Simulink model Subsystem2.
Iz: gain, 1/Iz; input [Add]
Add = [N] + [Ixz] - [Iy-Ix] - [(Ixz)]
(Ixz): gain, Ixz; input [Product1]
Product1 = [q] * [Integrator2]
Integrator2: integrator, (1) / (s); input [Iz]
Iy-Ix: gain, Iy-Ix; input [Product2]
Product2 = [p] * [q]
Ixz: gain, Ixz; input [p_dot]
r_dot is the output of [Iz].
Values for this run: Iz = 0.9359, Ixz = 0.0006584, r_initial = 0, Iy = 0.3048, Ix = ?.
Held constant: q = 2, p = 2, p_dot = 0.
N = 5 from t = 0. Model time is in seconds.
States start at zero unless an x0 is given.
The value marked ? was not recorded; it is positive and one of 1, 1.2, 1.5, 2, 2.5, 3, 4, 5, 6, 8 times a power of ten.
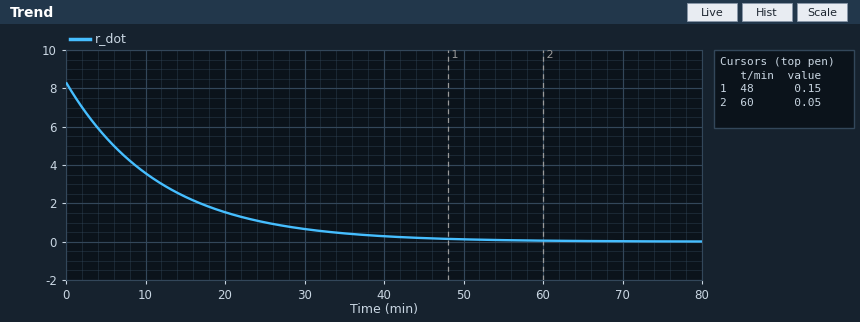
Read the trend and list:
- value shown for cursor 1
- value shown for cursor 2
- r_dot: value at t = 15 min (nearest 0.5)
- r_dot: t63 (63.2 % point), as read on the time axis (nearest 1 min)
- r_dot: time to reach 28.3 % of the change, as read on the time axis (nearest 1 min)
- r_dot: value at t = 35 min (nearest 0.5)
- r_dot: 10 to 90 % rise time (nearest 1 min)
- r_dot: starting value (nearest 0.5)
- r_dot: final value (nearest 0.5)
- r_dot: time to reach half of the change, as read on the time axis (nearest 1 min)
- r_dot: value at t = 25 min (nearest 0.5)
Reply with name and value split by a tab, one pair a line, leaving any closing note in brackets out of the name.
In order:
value shown for cursor 1	0.15
value shown for cursor 2	0.05
r_dot: value at t = 15 min	2.5
r_dot: t63 (63.2 % point), as read on the time axis	12 min
r_dot: time to reach 28.3 % of the change, as read on the time axis	4 min
r_dot: value at t = 35 min	0.5
r_dot: 10 to 90 % rise time	26 min
r_dot: starting value	8.5
r_dot: final value	0.0
r_dot: time to reach half of the change, as read on the time axis	8 min
r_dot: value at t = 25 min	1.0
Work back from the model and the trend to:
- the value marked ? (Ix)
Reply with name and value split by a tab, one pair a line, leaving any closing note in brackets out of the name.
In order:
the value marked ?	1
